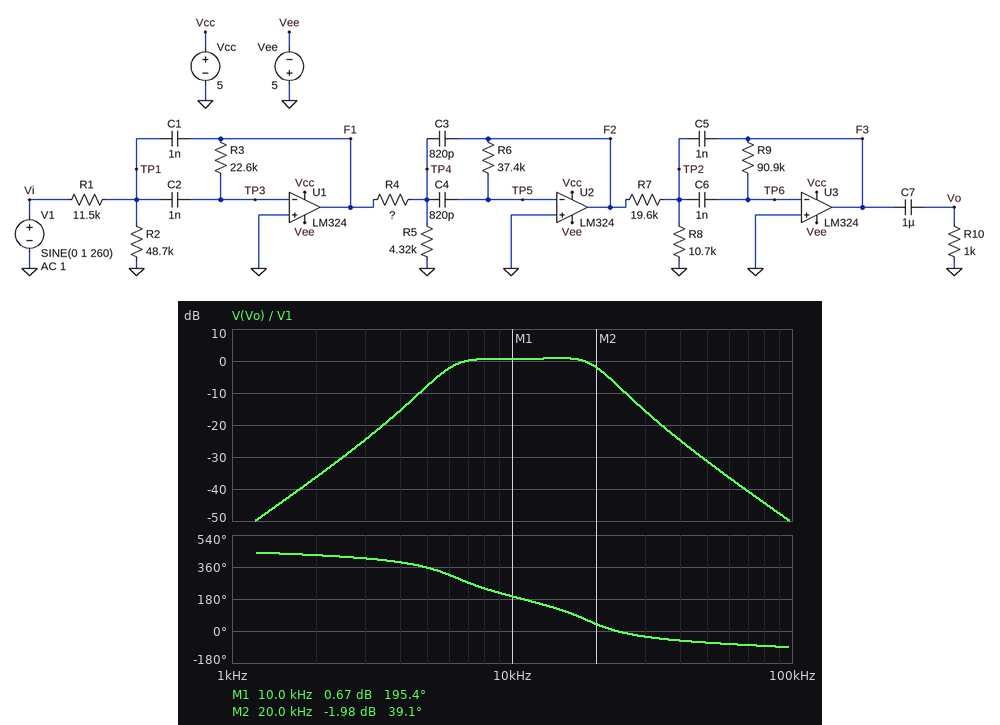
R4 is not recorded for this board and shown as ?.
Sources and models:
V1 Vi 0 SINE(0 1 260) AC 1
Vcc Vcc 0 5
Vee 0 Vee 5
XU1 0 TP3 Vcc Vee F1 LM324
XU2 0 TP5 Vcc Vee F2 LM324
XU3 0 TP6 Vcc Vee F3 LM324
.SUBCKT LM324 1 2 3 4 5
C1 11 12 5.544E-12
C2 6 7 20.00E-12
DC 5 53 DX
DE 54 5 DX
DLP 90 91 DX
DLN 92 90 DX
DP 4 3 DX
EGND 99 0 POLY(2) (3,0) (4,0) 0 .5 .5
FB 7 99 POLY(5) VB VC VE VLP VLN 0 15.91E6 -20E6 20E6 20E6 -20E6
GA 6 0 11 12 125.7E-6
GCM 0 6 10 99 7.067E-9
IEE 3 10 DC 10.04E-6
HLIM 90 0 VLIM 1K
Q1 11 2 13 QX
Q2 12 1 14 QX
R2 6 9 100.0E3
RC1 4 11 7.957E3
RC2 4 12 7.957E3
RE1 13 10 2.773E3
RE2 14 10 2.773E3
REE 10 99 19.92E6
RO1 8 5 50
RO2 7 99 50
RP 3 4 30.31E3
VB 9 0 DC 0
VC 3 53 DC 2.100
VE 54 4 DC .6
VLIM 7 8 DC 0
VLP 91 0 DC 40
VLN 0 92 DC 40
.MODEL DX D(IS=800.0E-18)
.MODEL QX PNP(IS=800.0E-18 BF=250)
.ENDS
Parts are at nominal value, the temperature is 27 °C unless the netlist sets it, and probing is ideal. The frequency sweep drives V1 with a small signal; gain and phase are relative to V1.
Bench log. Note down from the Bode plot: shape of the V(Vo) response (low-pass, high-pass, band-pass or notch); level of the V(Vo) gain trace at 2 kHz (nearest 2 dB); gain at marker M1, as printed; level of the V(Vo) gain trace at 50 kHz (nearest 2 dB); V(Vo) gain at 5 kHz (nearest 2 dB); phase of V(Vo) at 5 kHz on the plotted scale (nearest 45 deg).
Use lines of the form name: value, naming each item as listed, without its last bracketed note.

shape of the V(Vo) response: band-pass
level of the V(Vo) gain trace at 2 kHz: -36 dB
gain at marker M1, as printed: 0.67 dB
level of the V(Vo) gain trace at 50 kHz: -32 dB
V(Vo) gain at 5 kHz: -8 dB
phase of V(Vo) at 5 kHz on the plotted scale: 360 deg
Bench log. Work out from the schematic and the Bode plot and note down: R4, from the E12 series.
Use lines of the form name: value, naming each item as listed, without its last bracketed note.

R4, from the E12 series: 6.8 kΩ
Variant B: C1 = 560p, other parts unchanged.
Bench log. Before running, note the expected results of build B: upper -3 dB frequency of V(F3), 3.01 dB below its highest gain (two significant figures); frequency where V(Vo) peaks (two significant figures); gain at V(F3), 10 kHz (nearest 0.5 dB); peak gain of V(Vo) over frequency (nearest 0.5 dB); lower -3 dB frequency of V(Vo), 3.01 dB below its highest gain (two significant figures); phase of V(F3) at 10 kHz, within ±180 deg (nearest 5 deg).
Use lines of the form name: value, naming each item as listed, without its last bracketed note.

upper -3 dB frequency of V(F3), 3.01 dB below its highest gain: 21 kHz
frequency where V(Vo) peaks: 17 kHz
gain at V(F3), 10 kHz: 1.5 dB
peak gain of V(Vo) over frequency: 4.5 dB
lower -3 dB frequency of V(Vo), 3.01 dB below its highest gain: 9.1 kHz
phase of V(F3) at 10 kHz, within ±180 deg: -145 deg
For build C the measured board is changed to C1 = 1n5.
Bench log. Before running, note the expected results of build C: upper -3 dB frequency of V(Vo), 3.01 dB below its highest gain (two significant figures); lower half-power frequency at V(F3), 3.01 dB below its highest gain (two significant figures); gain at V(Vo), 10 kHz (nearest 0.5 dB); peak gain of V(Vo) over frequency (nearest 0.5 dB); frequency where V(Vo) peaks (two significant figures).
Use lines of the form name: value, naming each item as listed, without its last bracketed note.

upper -3 dB frequency of V(Vo), 3.01 dB below its highest gain: 18 kHz
lower half-power frequency at V(F3), 3.01 dB below its highest gain: 5.8 kHz
gain at V(Vo), 10 kHz: -1.5 dB
peak gain of V(Vo) over frequency: -0.5 dB
frequency where V(Vo) peaks: 7.5 kHz
